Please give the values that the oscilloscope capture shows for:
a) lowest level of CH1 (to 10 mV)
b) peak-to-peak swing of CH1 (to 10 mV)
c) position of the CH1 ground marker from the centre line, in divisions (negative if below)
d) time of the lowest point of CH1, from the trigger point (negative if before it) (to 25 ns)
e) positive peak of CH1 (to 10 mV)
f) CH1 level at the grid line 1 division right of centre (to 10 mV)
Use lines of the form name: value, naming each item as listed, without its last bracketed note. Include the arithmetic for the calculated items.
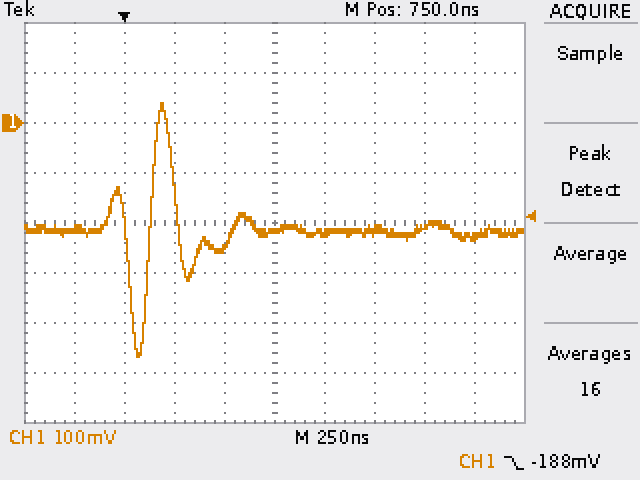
lowest level of CH1: -470 mV
peak-to-peak swing of CH1: 40 mV − (-470 mV) = 510 mV
position of the CH1 ground marker from the centre line, in divisions: +2.0 div
time of the lowest point of CH1, from the trigger point (negative if before it): +75 ns
positive peak of CH1: 40 mV
CH1 level at the grid line 1 division right of centre: -220 mV
